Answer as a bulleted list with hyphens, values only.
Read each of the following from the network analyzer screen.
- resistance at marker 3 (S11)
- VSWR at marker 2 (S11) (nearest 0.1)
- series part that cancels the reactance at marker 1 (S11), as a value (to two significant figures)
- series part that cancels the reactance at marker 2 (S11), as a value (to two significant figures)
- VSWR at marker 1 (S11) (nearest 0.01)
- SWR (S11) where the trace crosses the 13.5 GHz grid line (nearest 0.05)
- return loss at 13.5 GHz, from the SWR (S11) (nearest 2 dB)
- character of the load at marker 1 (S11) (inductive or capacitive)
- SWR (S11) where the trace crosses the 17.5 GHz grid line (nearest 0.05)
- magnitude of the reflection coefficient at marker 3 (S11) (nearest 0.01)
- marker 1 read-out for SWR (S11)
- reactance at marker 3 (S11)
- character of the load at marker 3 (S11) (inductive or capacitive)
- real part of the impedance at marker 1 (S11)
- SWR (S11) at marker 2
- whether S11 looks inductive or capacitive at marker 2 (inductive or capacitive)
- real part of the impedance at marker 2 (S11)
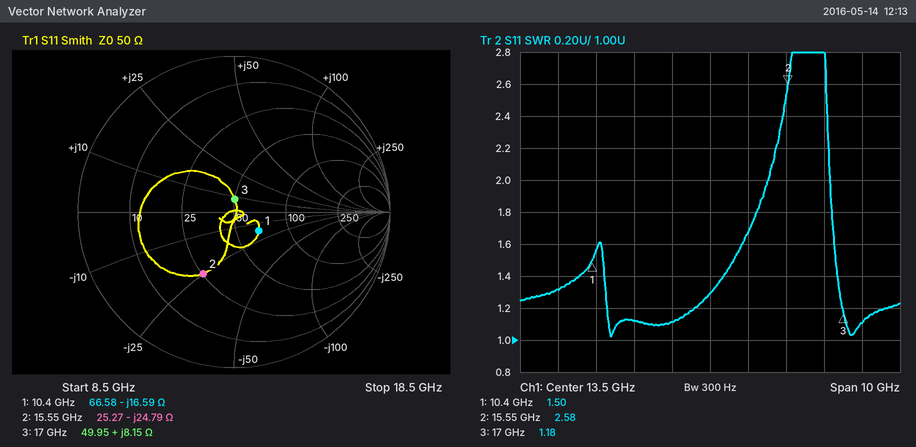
- 49.95 Ω
- 2.6
- 250 pH
- 250 pH
- 1.50
- 1.30
- 18 dB
- capacitive
- 1.10
- 0.08
- 1.50
- +8.15 Ω
- inductive
- 66.58 Ω
- 2.58
- capacitive
- 25.27 Ω
